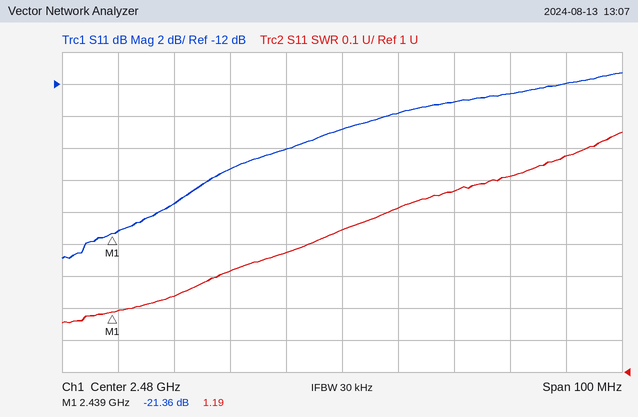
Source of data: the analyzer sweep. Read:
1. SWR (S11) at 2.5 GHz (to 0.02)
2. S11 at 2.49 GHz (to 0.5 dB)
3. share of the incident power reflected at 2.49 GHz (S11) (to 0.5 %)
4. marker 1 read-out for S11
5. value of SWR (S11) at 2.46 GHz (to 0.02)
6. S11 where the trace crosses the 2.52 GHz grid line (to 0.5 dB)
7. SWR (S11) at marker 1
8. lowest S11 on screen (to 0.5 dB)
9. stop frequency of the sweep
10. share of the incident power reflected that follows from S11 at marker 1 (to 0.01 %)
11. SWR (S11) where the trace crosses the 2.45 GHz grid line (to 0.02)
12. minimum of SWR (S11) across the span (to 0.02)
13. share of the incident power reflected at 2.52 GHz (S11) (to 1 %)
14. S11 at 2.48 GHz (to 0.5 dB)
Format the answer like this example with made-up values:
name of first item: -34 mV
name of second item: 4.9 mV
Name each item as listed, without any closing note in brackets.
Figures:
SWR (S11) at 2.5 GHz: 1.56
S11 at 2.49 GHz: -14.0 dB
share of the incident power reflected at 2.49 GHz (S11): 4.0 %
marker 1 read-out for S11: -21.36 dB
value of SWR (S11) at 2.46 GHz: 1.32
S11 where the trace crosses the 2.52 GHz grid line: -12.0 dB
SWR (S11) at marker 1: 1.19
lowest S11 on screen: -23.0 dB
stop frequency of the sweep: 2.53 GHz
share of the incident power reflected that follows from S11 at marker 1: 0.73 %
SWR (S11) where the trace crosses the 2.45 GHz grid line: 1.24
minimum of SWR (S11) across the span: 1.16
share of the incident power reflected at 2.52 GHz (S11): 6 %
S11 at 2.48 GHz: -15.0 dB
